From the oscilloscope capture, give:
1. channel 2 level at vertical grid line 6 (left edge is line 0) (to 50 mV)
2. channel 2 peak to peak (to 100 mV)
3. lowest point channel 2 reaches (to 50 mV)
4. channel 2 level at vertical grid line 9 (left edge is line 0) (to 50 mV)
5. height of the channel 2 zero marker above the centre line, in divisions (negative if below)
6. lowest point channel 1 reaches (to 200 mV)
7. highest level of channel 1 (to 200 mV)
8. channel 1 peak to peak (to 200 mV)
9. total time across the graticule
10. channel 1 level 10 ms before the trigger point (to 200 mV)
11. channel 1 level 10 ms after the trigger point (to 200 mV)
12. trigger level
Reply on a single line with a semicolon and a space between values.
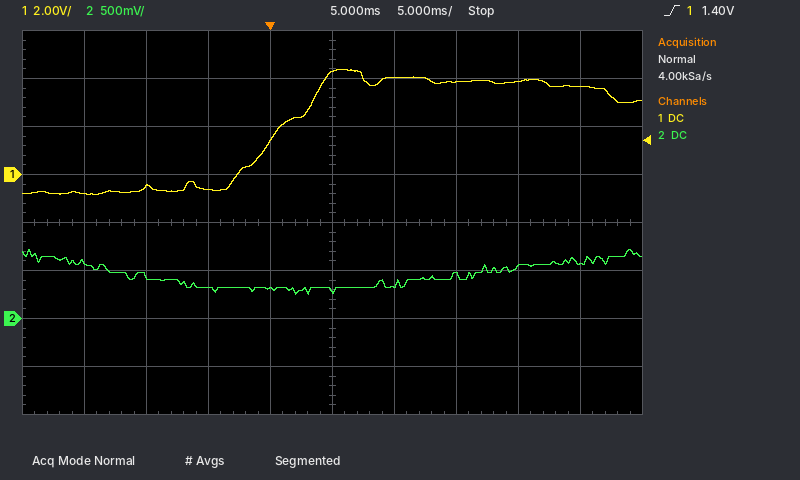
350 mV; 500 mV; 250 mV; 550 mV; -2.0 div; -800 mV; 4.4 V; 5.2 V; 50 ms; -600 mV; 4.0 V; 1.40 V
